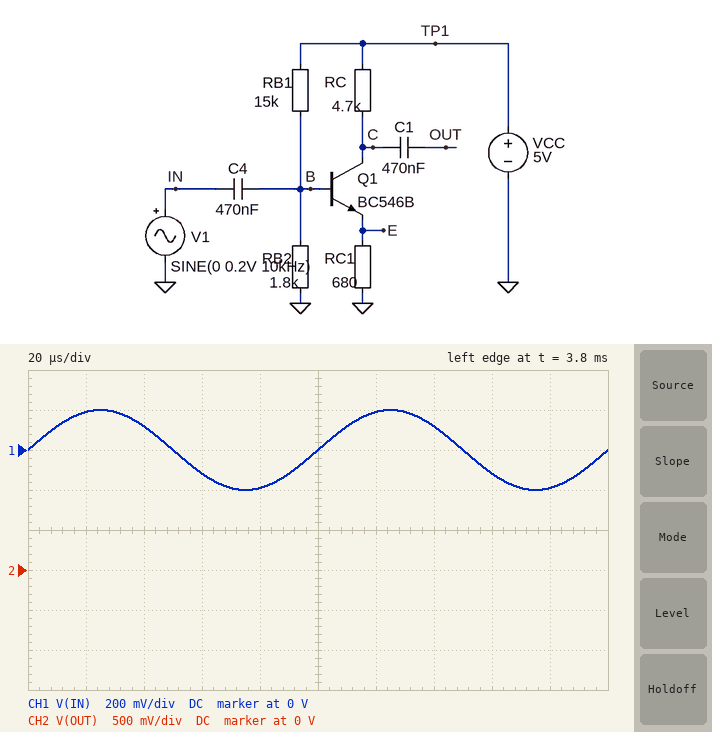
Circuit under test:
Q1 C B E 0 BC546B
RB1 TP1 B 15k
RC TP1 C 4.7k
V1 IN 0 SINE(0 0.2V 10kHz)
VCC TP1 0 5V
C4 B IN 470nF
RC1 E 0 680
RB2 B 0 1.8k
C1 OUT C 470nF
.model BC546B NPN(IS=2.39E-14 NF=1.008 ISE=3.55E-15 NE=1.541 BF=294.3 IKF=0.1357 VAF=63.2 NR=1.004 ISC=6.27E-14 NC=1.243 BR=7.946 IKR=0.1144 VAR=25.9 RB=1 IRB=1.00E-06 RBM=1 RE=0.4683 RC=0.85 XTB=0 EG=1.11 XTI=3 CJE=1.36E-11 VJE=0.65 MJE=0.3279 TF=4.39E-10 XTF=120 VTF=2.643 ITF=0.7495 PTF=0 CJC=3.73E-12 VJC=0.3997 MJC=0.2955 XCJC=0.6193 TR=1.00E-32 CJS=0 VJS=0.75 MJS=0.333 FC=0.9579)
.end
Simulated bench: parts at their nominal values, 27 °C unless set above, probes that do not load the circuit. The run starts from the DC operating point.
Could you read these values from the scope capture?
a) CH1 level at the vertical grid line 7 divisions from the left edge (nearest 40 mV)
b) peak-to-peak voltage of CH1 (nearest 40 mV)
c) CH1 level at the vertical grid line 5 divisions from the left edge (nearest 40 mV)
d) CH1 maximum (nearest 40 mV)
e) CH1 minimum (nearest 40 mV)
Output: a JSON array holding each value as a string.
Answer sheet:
["120 mV", "400 mV", "0 V", "200 mV", "-200 mV"]
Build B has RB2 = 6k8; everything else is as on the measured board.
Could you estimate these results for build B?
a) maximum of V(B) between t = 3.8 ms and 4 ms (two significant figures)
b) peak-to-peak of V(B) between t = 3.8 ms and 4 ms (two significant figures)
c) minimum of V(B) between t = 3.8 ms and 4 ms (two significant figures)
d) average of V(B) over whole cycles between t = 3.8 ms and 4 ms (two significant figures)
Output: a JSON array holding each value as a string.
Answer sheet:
["1.4 V", "400 mV", "1.0 V", "1.2 V"]
